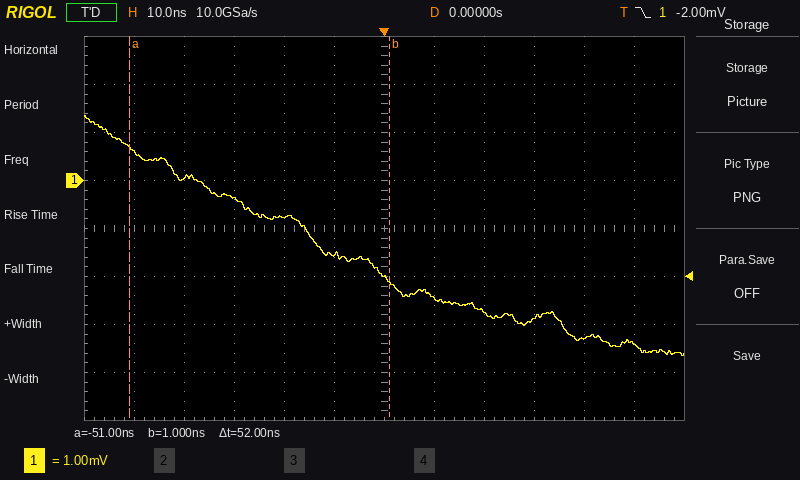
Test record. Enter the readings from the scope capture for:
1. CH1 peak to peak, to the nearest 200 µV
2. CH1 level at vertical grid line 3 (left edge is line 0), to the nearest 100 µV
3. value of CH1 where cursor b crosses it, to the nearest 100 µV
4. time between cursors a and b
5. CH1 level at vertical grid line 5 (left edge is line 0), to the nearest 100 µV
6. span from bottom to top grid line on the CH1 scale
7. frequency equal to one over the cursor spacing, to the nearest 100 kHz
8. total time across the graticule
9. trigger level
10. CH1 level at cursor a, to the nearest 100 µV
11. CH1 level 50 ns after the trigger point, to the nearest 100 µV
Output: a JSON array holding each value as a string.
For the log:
["5.0 mV", "-400 µV", "-2.1 mV", "52 ns", "-1.5 mV", "8 mV", "19.2 MHz", "120 ns", "-2.00 mV", "700 µV", "-3.4 mV"]
